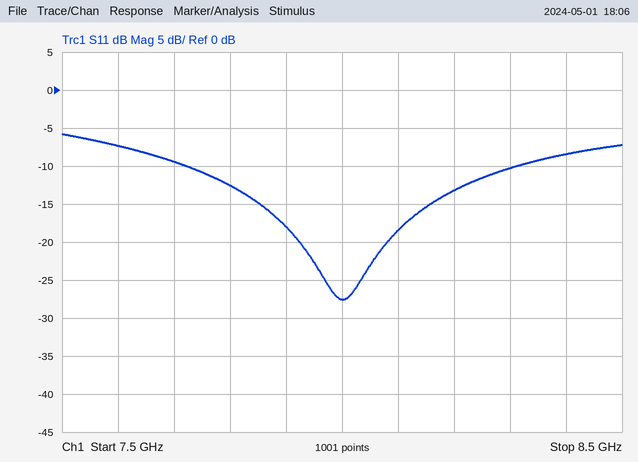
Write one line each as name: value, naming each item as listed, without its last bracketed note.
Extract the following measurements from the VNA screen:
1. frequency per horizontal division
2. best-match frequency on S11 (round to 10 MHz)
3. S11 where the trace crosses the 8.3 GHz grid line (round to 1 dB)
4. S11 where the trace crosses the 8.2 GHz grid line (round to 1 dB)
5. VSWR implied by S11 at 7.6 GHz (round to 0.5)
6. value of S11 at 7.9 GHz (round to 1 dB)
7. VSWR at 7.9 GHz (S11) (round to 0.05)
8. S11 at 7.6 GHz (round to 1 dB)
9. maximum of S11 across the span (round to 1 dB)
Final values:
frequency per horizontal division: 100 MHz
best-match frequency on S11: 8.00 GHz
S11 where the trace crosses the 8.3 GHz grid line: -10 dB
S11 where the trace crosses the 8.2 GHz grid line: -13 dB
VSWR implied by S11 at 7.6 GHz: 2.5
value of S11 at 7.9 GHz: -18 dB
VSWR at 7.9 GHz (S11): 1.30
S11 at 7.6 GHz: -7 dB
maximum of S11 across the span: -6 dB
